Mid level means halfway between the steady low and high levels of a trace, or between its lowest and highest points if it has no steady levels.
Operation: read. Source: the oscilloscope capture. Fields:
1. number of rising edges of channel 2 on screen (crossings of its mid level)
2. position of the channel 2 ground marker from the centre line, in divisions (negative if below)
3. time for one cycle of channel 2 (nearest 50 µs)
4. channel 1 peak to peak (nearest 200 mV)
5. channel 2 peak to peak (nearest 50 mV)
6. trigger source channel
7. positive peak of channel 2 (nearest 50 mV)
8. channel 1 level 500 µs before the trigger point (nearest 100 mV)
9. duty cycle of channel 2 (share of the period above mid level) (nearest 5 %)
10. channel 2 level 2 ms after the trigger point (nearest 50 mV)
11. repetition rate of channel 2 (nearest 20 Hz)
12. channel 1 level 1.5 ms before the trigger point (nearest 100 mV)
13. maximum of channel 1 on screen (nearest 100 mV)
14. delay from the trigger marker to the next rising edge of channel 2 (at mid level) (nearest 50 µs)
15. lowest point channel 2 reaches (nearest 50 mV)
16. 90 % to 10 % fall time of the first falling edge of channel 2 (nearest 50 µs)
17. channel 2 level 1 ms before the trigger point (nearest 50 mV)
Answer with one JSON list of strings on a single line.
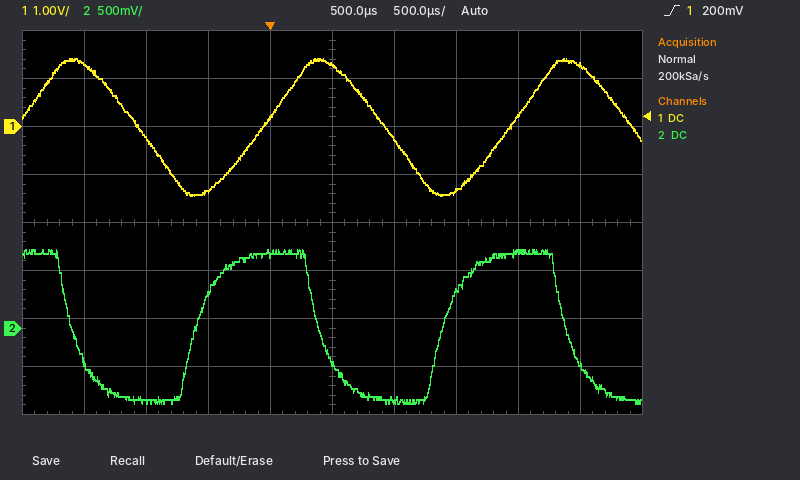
["2", "-2.2 div", "2.00 ms", "2.8 V", "1.60 V", "channel 1", "800 mV", "-1.3 V", "50 %", "800 mV", "500 Hz", "1.3 V", "1.4 V", "1.40 ms", "-800 mV", "350 µs", "-750 mV"]
